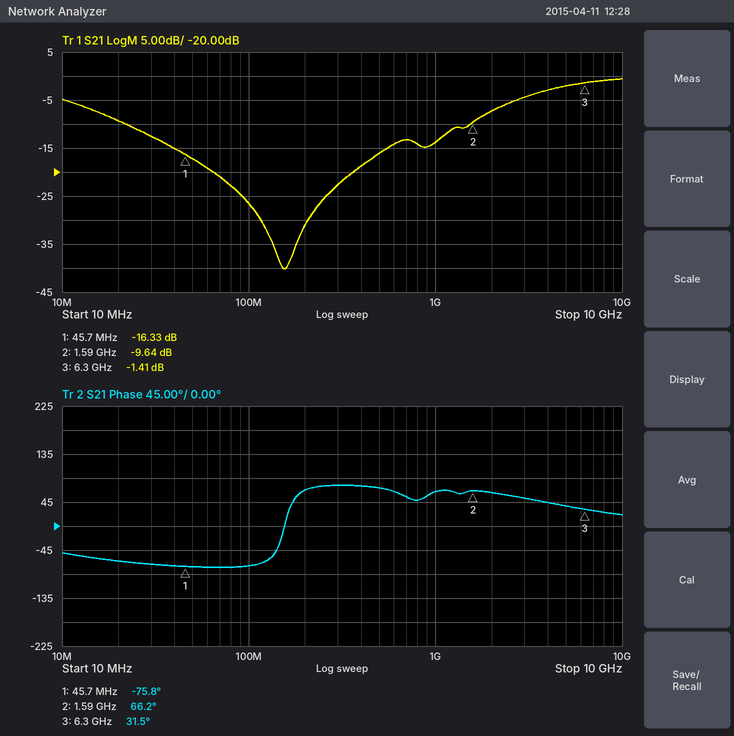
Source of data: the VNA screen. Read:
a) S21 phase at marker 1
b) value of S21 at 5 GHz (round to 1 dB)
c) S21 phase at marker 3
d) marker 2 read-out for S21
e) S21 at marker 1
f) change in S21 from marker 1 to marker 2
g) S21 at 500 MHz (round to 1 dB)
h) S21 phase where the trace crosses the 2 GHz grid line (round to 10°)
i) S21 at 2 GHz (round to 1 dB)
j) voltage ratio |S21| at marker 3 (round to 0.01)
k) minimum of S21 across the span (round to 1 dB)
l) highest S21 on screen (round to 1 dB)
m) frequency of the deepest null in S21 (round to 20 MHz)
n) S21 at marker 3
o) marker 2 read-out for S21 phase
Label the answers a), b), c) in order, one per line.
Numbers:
a) -75.8°
b) -2 dB
c) 31.5°
d) -9.64 dB
e) -16.33 dB
f) 6.69 dB
g) -16 dB
h) 60°
i) -7 dB
j) 0.85
k) -40 dB
l) -1 dB
m) 160 MHz
n) -1.41 dB
o) 66.2°
